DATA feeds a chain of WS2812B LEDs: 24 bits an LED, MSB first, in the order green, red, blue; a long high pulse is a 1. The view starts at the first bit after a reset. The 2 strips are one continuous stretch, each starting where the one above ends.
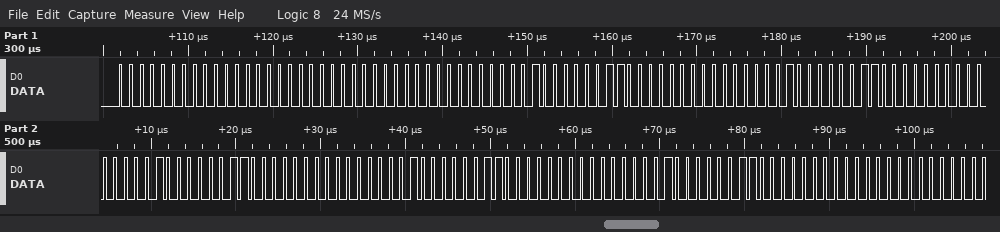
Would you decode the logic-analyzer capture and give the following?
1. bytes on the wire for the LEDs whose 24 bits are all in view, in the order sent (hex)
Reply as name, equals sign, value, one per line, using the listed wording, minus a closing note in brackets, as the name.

bytes on the wire for the LEDs whose 24 bits are all in view, in the order sent = 00 00 00 00 01 03 00 01 03 00 01 03 00 01 03 00 01 03
